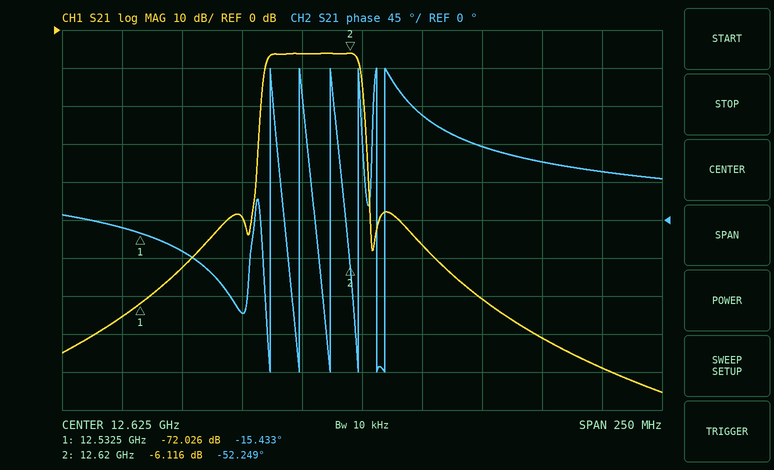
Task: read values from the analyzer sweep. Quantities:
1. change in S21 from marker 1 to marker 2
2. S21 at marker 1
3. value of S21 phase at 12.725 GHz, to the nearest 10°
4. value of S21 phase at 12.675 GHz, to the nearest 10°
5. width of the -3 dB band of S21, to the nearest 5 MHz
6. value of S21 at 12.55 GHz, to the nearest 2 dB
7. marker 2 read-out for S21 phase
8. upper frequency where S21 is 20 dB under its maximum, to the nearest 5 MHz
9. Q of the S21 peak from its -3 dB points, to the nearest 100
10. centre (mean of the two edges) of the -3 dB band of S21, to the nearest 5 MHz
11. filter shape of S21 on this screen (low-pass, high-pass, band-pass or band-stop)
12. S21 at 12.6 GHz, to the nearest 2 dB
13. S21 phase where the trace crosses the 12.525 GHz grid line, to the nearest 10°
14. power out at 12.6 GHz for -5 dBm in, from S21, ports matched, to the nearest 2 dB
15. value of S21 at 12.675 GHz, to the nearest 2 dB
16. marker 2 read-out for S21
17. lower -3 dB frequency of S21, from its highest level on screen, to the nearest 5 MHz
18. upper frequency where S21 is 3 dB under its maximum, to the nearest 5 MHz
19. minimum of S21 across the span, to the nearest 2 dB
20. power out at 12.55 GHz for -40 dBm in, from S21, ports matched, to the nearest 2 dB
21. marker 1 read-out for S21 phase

65.910 dB
-72.026 dB
60°
90°
40 MHz
-62 dB
-52.249°
12.625 GHz
300
12.605 GHz
band-pass
-6 dB
-10°
-12 dBm
-70 dB
-6.116 dB
12.585 GHz
12.625 GHz
-96 dB
-102 dBm
-15.433°
